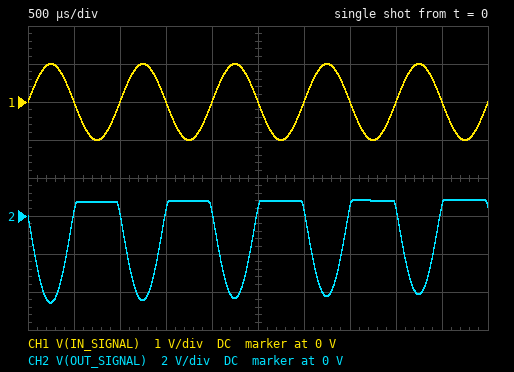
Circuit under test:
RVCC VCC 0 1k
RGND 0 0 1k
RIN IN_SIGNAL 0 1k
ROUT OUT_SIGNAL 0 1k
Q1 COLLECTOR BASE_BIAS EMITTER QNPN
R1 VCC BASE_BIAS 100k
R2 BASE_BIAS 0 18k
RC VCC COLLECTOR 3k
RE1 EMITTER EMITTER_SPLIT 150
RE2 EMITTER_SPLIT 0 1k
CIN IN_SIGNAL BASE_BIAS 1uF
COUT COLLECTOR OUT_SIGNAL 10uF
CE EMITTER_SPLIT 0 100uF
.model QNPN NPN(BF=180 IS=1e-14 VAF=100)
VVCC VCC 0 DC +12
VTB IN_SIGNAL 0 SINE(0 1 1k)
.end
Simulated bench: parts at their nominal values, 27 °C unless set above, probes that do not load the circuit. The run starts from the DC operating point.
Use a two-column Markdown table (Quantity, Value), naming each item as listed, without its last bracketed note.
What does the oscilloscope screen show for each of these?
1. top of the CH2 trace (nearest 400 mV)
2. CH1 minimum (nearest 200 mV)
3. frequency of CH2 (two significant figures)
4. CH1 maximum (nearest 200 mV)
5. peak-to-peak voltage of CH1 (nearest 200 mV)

| Quantity | Value |
|---|---|
| top of the CH2 trace | 800 mV |
| CH1 minimum | -1.0 V |
| frequency of CH2 | 1.0 kHz |
| CH1 maximum | 1.0 V |
| peak-to-peak voltage of CH1 | 2.0 V |
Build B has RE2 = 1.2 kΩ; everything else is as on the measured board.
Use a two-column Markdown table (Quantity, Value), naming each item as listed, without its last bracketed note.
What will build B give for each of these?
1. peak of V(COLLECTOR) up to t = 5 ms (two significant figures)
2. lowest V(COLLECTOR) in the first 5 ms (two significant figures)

| Quantity | Value |
|---|---|
| peak of V(COLLECTOR) up to t = 5 ms | 10 V |
| lowest V(COLLECTOR) in the first 5 ms | 4.9 V |
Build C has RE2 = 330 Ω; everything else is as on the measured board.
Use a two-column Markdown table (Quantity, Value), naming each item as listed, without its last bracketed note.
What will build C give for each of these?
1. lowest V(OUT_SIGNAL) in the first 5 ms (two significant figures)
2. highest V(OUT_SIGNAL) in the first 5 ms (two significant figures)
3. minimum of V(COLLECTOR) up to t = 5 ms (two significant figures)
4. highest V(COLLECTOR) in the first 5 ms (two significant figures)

| Quantity | Value |
|---|---|
| lowest V(OUT_SIGNAL) in the first 5 ms | -3.9 V |
| highest V(OUT_SIGNAL) in the first 5 ms | 1.6 V |
| minimum of V(COLLECTOR) up to t = 5 ms | 1.9 V |
| highest V(COLLECTOR) in the first 5 ms | 7.3 V |
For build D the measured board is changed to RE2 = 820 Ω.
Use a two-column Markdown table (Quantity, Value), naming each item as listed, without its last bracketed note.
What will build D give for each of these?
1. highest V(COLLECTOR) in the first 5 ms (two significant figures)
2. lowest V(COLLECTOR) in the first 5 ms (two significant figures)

| Quantity | Value |
|---|---|
| highest V(COLLECTOR) in the first 5 ms | 9.4 V |
| lowest V(COLLECTOR) in the first 5 ms | 4.0 V |
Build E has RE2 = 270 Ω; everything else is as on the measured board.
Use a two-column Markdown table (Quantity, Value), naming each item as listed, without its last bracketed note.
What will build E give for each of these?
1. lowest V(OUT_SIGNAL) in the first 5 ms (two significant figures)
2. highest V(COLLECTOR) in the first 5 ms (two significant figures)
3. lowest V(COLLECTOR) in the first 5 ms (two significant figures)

| Quantity | Value |
|---|---|
| lowest V(OUT_SIGNAL) in the first 5 ms | -3.3 V |
| highest V(COLLECTOR) in the first 5 ms | 6.8 V |
| lowest V(COLLECTOR) in the first 5 ms | 1.8 V |
